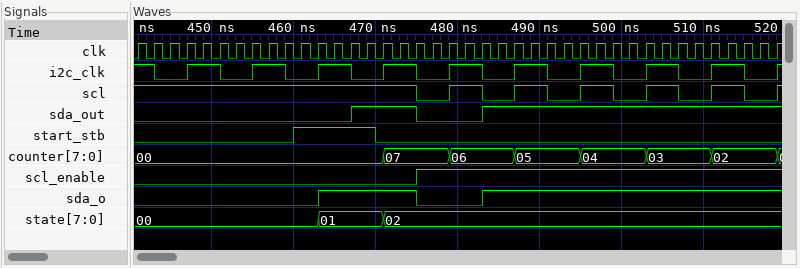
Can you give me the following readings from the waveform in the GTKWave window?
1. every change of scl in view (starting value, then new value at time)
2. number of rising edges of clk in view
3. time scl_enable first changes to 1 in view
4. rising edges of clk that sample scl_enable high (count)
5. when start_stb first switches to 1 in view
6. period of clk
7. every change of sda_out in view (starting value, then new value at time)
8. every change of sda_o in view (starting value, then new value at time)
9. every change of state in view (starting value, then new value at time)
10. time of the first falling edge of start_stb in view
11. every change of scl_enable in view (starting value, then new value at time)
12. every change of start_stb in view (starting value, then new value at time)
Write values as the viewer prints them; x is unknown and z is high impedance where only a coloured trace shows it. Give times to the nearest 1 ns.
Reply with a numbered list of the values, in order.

1. 1, 0 at 475 ns, 1 at 479 ns, 0 at 483 ns, 1 at 487 ns, 0 at 491 ns, 1 at 495 ns, 0 at 499 ns, 1 at 503 ns, 0 at 507 ns, 1 at 511 ns, 0 at 515 ns, 1 at 519 ns
2. 40
3. 475 ns
4. 22
5. 460 ns
6. 2 ns
7. 0, 1 at 467 ns, 0 at 475 ns, 1 at 483 ns
8. 0, 1 at 463 ns, 0 at 475 ns, 1 at 483 ns
9. 00, 01 at 463 ns, 02 at 471 ns
10. 470 ns
11. 0, 1 at 475 ns
12. 0, 1 at 460 ns, 0 at 470 ns
